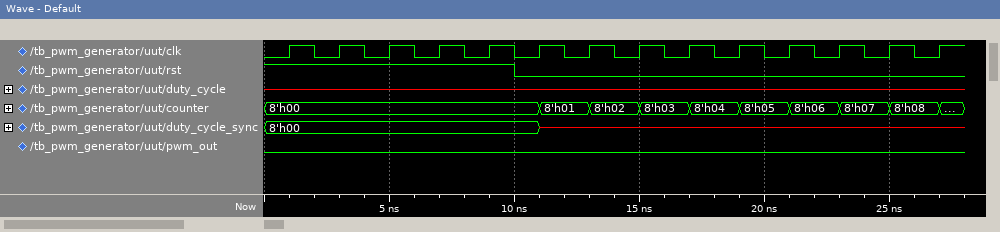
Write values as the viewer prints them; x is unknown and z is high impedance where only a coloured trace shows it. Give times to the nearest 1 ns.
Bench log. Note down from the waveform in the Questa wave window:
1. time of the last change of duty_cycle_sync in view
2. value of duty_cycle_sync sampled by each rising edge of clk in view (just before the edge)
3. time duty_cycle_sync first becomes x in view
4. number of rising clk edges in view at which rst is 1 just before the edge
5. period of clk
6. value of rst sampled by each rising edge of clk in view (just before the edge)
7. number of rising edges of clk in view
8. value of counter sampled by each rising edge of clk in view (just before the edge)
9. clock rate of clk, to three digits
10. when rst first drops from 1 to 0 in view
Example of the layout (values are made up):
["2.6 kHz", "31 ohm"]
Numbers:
["11 ns", "8'h00, 8'h00, 8'h00, 8'h00, 8'h00, 8'h00, x, x, x, x, x, x, x, x", "11 ns", "5", "2 ns", "1 1 1 1 1 0 0 0 0 0 0 0 0 0", "14", "8'h00, 8'h00, 8'h00, 8'h00, 8'h00, 8'h00, 8'h01, 8'h02, 8'h03, 8'h04, 8'h05, 8'h06, 8'h07, 8'h08", "500 MHz", "10 ns"]
